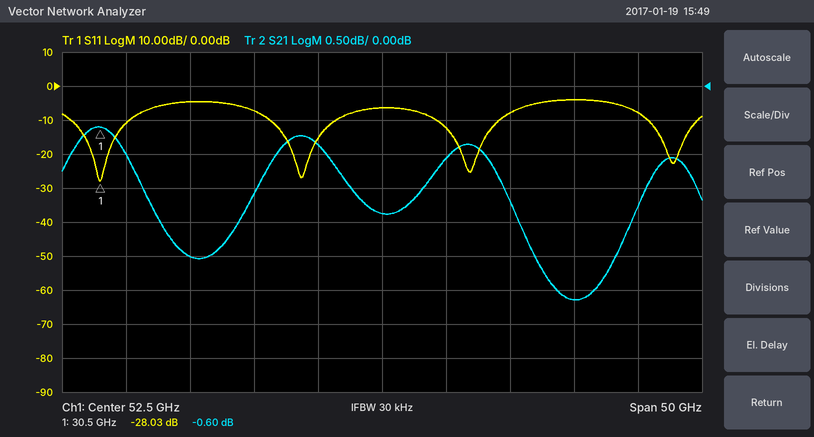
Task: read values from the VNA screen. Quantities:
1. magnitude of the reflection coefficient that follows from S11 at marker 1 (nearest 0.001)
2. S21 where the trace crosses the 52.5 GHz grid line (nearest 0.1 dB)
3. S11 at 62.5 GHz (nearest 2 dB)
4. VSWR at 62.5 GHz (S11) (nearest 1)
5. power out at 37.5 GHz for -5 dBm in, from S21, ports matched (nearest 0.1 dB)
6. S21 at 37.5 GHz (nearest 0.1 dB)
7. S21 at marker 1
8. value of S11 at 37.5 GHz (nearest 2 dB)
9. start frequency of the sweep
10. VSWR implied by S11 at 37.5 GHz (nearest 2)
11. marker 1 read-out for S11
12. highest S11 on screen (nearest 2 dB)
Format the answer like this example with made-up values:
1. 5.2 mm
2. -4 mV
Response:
1. 0.040
2. -1.9 dB
3. -8 dB
4. 2
5. -7.5 dBm
6. -2.5 dB
7. -0.60 dB
8. -4 dB
9. 27.5 GHz
10. 4
11. -28.03 dB
12. -4 dB
